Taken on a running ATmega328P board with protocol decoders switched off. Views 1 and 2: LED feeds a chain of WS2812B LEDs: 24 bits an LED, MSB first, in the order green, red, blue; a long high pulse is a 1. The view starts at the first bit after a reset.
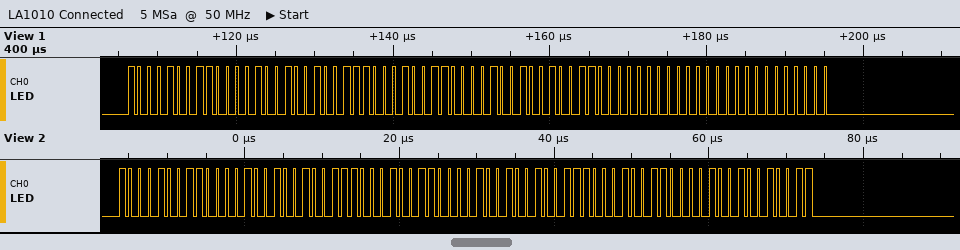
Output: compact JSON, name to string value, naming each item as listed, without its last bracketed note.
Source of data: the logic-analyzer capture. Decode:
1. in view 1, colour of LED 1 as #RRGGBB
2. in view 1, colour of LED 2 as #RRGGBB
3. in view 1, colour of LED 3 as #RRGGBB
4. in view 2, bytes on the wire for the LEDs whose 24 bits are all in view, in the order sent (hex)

{"in view 1, colour of LED 1 as #RRGGBB": "#848993", "in view 1, colour of LED 2 as #RRGGBB": "#848993", "in view 1, colour of LED 3 as #RRGGBB": "#000000", "in view 2, bytes on the wire for the LEDs whose 24 bits are all in view, in the order sent": "89 84 93 89 84 93 89 84 93"}
